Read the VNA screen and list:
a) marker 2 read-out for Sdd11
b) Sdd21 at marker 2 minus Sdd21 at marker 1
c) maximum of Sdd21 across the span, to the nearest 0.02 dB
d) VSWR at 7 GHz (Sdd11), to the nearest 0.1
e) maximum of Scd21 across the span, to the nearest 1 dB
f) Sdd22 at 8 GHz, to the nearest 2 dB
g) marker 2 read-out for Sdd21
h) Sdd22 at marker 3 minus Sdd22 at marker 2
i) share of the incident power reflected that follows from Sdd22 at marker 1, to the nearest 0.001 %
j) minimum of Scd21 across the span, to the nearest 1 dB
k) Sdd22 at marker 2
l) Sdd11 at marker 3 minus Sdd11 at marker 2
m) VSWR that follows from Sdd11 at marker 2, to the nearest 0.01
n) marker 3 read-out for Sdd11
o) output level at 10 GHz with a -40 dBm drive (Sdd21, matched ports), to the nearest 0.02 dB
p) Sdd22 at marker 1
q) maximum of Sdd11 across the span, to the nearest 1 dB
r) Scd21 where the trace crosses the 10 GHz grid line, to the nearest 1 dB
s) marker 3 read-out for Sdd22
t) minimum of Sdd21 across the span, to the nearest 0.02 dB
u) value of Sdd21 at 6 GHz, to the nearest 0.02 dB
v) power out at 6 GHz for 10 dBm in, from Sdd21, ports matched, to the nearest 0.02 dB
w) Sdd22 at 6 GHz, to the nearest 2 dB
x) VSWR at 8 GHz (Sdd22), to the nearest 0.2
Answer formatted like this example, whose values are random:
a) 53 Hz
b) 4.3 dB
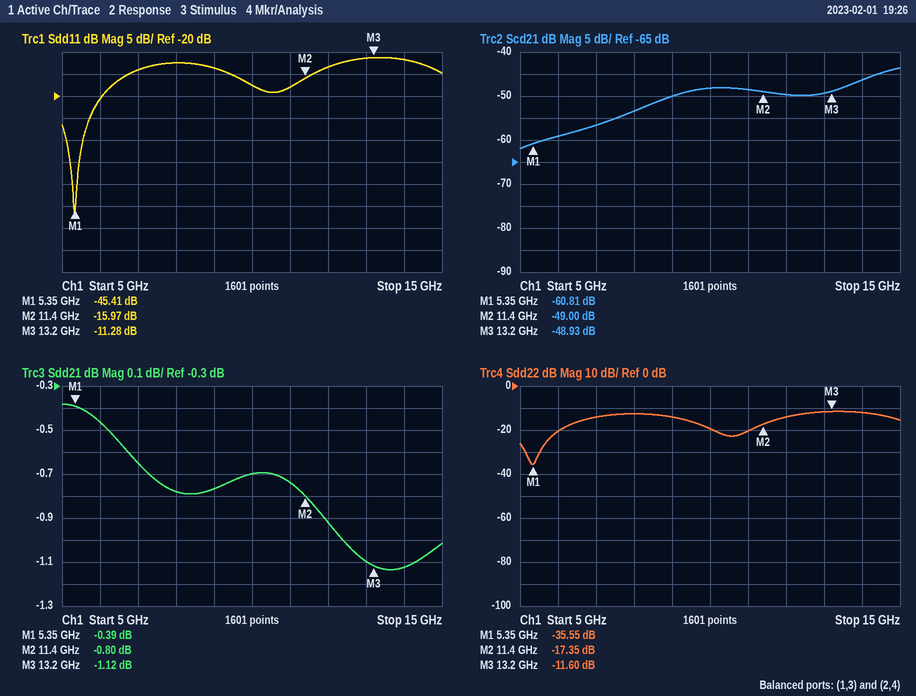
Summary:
a) -15.97 dB
b) -0.41 dB
c) -0.38 dB
d) 1.5
e) -44 dB
f) -12 dB
g) -0.80 dB
h) 5.75 dB
i) 0.028 %
j) -62 dB
k) -17.35 dB
l) 4.69 dB
m) 1.38
n) -11.28 dB
o) -40.70 dBm
p) -35.55 dB
q) -11 dB
r) -48 dB
s) -11.60 dB
t) -1.14 dB
u) -0.46 dB
v) 9.54 dBm
w) -20 dB
x) 1.6
